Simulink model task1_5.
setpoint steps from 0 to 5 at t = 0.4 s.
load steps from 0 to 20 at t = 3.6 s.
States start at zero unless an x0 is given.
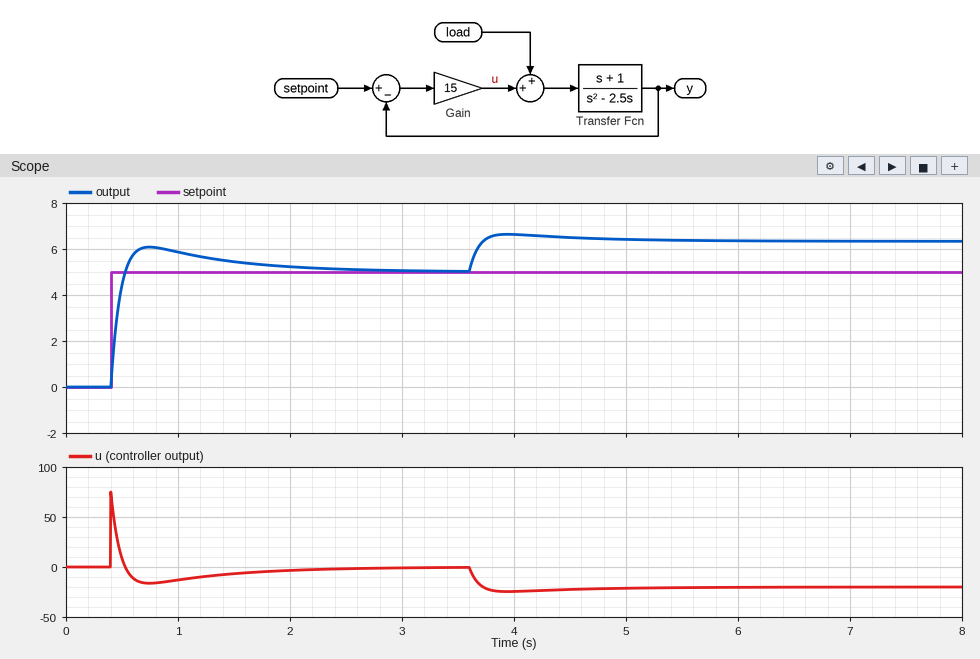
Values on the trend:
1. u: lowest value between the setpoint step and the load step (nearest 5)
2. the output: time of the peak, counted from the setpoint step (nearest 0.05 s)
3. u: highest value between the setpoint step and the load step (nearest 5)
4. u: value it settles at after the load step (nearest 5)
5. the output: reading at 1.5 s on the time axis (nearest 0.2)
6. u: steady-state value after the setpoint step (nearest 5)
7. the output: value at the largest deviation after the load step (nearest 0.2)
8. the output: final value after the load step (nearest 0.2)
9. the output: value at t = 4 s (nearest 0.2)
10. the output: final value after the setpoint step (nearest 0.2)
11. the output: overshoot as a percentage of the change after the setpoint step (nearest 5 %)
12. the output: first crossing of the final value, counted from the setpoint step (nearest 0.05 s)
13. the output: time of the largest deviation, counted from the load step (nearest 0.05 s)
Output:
-15
0.35 s
75
-20
5.4
0
6.6
6.4
6.6
5.0
20 %
0.15 s
0.35 s
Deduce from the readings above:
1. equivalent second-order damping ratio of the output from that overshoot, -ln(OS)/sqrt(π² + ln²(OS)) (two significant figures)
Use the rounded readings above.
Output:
0.46
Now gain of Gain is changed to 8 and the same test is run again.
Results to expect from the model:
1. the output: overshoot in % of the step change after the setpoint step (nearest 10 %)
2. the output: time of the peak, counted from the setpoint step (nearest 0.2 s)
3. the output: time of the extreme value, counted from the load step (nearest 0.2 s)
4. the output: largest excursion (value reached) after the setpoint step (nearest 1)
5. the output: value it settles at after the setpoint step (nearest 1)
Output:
40 %
0.6 s
0.6 s
7
5
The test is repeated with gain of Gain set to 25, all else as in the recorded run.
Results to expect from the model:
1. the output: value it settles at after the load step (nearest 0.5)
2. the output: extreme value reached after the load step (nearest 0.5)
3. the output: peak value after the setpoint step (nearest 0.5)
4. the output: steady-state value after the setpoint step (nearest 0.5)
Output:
6.0
6.0
5.5
5.0
